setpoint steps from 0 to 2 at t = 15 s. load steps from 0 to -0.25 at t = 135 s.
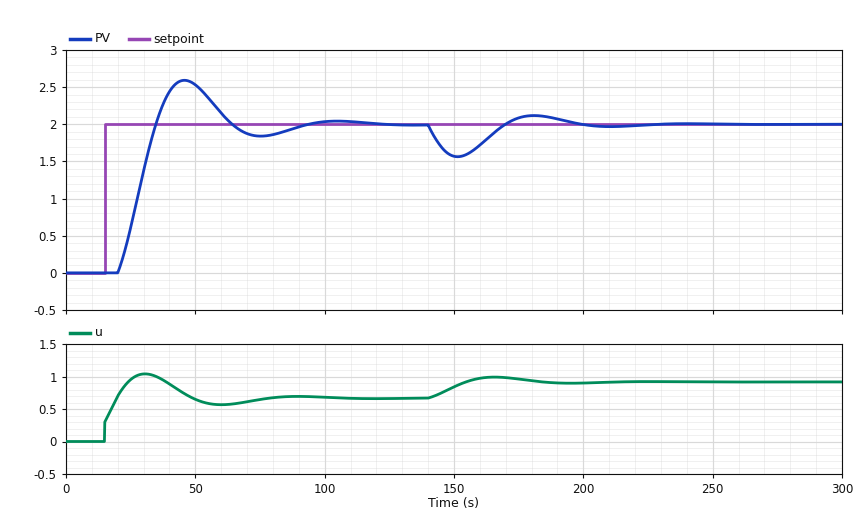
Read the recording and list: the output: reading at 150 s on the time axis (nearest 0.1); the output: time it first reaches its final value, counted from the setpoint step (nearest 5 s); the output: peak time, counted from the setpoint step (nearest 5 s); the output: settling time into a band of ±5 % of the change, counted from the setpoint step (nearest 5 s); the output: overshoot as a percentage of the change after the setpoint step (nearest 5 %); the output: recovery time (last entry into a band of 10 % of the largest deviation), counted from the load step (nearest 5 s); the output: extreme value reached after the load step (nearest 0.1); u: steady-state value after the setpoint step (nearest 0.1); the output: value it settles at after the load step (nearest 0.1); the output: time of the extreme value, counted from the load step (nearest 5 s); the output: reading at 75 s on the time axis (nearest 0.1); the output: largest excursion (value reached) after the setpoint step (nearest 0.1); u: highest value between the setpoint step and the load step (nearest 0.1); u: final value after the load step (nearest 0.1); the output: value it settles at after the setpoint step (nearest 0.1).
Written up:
1.6
20 s
30 s
70 s
30 %
60 s
1.6
0.7
2.0
15 s
1.8
2.6
1.0
0.9
2.0
